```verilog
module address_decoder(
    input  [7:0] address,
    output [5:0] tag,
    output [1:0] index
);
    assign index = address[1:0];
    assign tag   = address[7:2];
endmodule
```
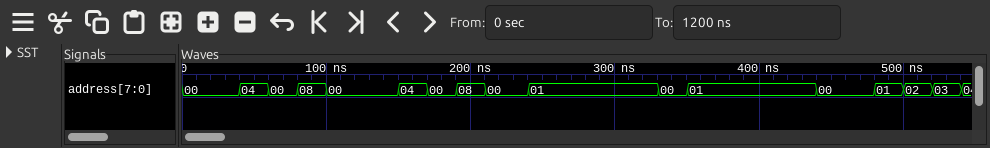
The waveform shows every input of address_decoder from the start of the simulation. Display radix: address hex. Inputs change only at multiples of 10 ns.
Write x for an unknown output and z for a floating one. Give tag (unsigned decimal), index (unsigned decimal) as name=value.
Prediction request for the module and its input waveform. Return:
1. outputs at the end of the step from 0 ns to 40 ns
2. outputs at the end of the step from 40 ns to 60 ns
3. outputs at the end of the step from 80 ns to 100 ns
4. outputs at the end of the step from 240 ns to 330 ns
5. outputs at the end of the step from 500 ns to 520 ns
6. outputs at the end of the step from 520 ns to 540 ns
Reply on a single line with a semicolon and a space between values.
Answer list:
tag=0, index=0; tag=1, index=0; tag=2, index=0; tag=0, index=1; tag=0, index=2; tag=0, index=3
